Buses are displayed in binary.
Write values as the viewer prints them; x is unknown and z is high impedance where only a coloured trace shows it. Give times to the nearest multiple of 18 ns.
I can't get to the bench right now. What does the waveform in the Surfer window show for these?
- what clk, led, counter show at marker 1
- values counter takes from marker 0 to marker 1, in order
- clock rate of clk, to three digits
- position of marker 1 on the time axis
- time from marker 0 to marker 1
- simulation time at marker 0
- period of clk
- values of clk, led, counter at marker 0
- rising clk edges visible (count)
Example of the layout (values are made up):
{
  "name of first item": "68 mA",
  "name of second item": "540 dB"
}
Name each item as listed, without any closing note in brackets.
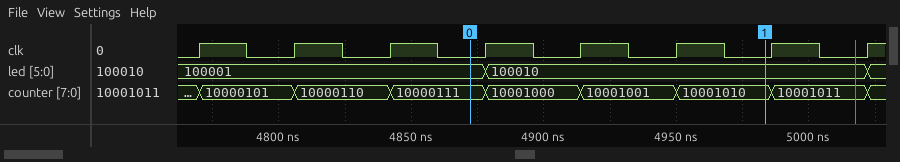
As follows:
{
  "what clk, led, counter show at marker 1": "clk=0, led=100010, counter=10001010",
  "values counter takes from marker 0 to marker 1, in order": "10000111, 10001000, 10001001, 10001010",
  "clock rate of clk, to three digits": "27.8 MHz",
  "position of marker 1 on the time axis": "4986 ns",
  "time from marker 0 to marker 1": "108 ns",
  "simulation time at marker 0": "4878 ns",
  "period of clk": "36 ns",
  "values of clk, led, counter at marker 0": "clk=0, led=100001, counter=10000111",
  "rising clk edges visible": "8"
}
